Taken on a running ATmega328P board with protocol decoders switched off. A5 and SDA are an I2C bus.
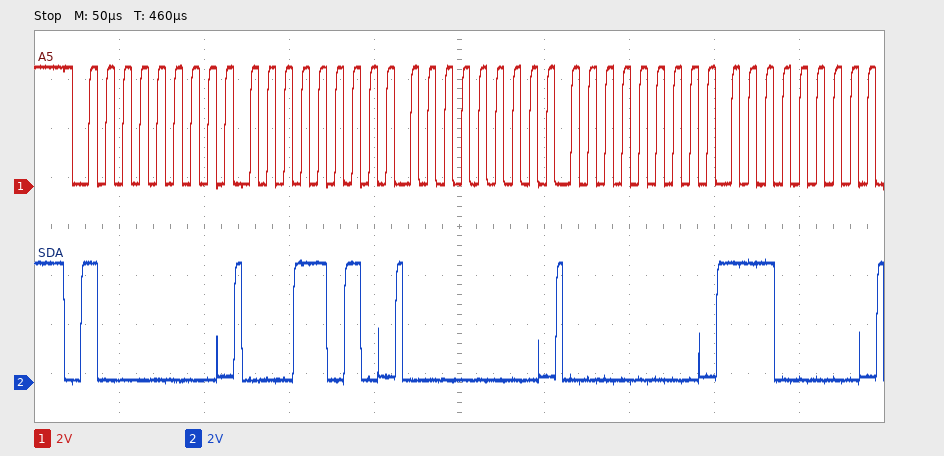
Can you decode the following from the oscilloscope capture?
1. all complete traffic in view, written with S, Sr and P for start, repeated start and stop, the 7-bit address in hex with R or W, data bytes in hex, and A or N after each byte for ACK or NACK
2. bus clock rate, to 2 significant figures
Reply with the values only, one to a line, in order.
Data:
S 40W A 1A A 00 A 00 A E0 A
100 kHz
